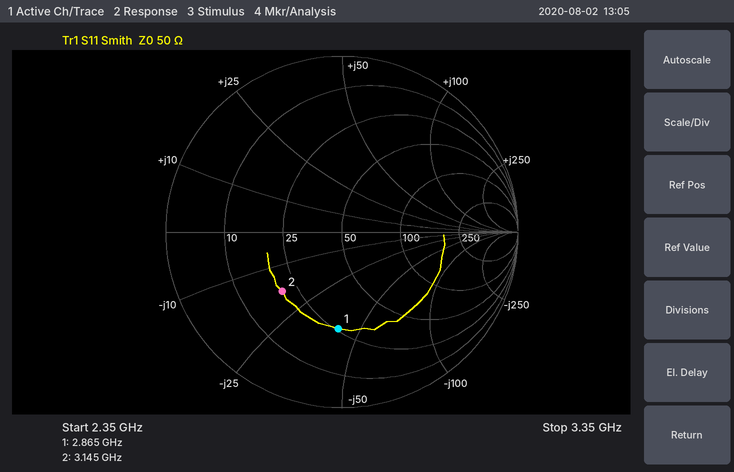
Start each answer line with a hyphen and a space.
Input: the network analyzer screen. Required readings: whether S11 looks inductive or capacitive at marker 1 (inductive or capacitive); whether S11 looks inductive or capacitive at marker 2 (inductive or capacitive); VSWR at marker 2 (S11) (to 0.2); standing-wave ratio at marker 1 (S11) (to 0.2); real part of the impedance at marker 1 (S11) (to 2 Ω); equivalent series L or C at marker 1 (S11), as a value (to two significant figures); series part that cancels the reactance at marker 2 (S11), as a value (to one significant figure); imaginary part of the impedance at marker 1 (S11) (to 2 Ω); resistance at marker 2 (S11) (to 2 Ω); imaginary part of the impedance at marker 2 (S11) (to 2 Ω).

- capacitive
- capacitive
- 2.8
- 3.4
- 26 Ω
- 1.4 pF
- 900 pH
- -40 Ω
- 20 Ω
- -18 Ω
